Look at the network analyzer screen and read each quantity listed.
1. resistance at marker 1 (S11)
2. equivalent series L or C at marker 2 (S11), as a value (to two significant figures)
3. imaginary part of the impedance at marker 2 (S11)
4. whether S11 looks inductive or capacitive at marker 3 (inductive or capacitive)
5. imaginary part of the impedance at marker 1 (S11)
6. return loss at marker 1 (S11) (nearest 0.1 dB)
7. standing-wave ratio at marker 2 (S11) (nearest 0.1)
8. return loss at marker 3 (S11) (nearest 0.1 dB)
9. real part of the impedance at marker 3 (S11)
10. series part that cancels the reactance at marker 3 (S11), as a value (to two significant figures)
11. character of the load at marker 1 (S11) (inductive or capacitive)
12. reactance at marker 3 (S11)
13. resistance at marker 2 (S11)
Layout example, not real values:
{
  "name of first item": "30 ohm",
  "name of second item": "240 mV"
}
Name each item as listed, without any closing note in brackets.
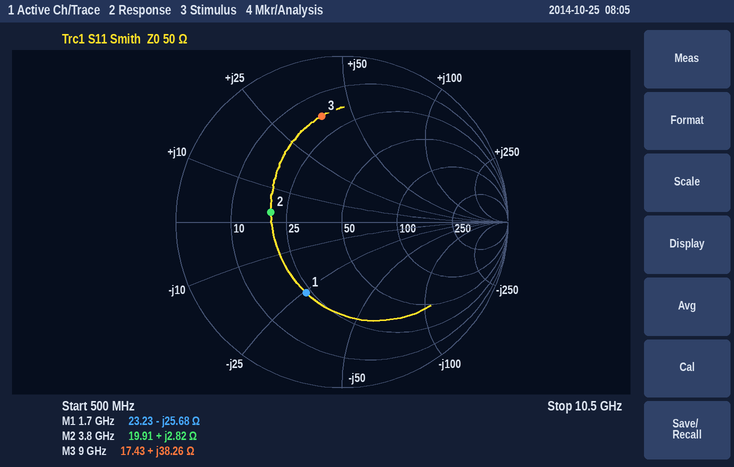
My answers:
{
  "resistance at marker 1": "23.23 Ω",
  "equivalent series L or C at marker 2 (S11), as a value": "120 pH",
  "imaginary part of the impedance at marker 2": "+2.82 Ω",
  "whether S11 looks inductive or capacitive at marker 3": "inductive",
  "imaginary part of the impedance at marker 1": "-25.68 Ω",
  "return loss at marker 1 (S11)": "6.4 dB",
  "standing-wave ratio at marker 2 (S11)": "2.5",
  "return loss at marker 3 (S11)": "3.8 dB",
  "real part of the impedance at marker 3": "17.43 Ω",
  "series part that cancels the reactance at marker 3 (S11), as a value": "460 fF",
  "character of the load at marker 1 (S11)": "capacitive",
  "reactance at marker 3": "+38.26 Ω",
  "resistance at marker 2": "19.91 Ω"
}
